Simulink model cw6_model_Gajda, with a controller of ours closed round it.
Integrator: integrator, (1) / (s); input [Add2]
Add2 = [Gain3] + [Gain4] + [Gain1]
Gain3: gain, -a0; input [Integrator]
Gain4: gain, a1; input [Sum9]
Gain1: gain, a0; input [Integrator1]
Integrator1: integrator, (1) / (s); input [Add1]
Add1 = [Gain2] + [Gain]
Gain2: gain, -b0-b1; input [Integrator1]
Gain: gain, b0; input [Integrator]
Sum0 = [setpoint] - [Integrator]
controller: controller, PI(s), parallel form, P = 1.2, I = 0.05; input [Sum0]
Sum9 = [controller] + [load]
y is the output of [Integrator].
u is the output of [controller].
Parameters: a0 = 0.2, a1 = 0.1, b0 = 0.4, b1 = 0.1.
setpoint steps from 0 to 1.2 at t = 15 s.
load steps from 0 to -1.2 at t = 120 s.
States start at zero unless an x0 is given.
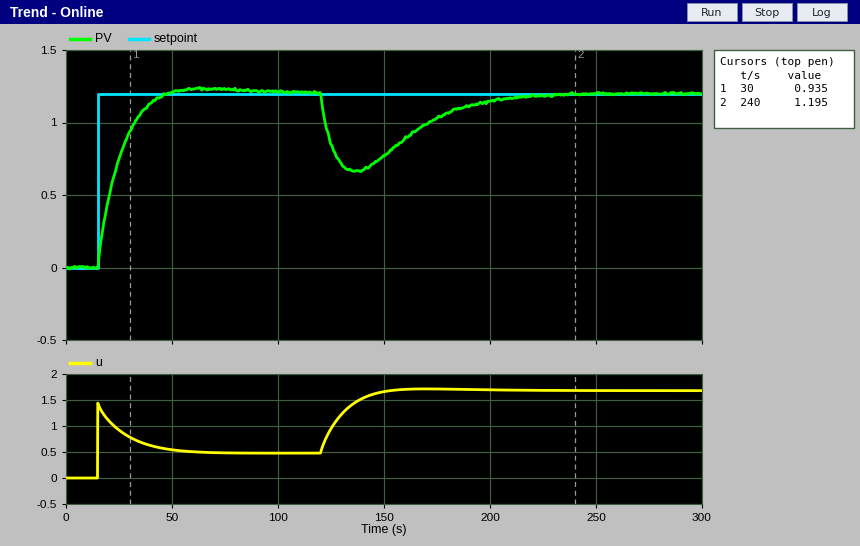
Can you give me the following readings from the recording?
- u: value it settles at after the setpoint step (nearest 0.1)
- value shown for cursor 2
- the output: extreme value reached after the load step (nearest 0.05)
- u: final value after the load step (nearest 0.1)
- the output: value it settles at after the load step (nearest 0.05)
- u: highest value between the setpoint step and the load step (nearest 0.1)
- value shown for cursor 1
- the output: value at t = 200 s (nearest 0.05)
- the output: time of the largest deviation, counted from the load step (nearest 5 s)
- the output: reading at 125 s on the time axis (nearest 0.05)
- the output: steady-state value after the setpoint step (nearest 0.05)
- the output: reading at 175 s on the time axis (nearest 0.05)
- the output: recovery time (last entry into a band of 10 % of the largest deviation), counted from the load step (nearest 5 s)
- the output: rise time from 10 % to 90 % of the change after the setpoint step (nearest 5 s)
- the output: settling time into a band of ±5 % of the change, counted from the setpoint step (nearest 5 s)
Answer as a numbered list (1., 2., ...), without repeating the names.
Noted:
1. 0.5
2. 1.195
3. 0.65
4. 1.7
5. 1.20
6. 1.4
7. 0.935
8. 1.15
9. 15 s
10. 0.85
11. 1.20
12. 1.05
13. 80 s
14. 20 s
15. 25 s
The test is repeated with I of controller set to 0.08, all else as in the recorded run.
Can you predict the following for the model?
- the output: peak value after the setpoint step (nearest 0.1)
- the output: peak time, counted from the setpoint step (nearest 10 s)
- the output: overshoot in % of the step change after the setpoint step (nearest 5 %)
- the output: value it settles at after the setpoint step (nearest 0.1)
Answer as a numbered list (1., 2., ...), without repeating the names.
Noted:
1. 1.3
2. 40 s
3. 10 %
4. 1.2
